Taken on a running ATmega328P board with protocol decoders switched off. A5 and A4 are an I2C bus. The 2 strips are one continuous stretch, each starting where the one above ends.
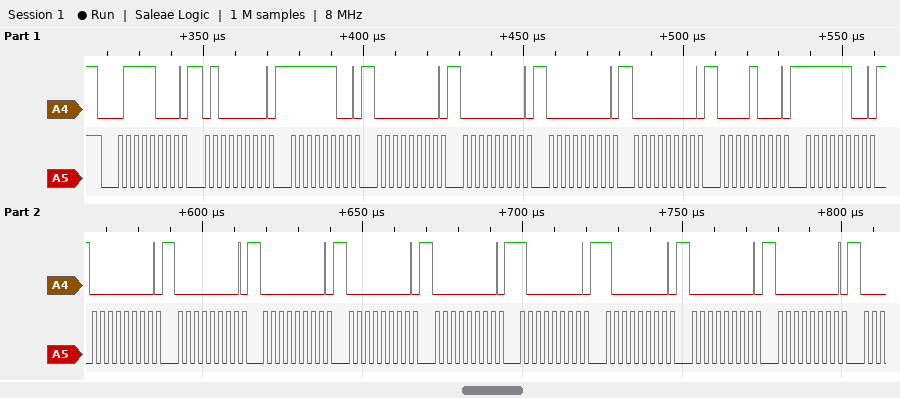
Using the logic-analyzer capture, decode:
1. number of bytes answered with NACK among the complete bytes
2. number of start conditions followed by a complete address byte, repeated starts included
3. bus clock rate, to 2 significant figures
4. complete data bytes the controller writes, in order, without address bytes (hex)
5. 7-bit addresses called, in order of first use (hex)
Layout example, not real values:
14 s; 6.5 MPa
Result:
0; 1; 400 kHz; 40 FC 00 00 00 00 08 FC 00 00 00 00 00 80 80 00 00; 0x3C
